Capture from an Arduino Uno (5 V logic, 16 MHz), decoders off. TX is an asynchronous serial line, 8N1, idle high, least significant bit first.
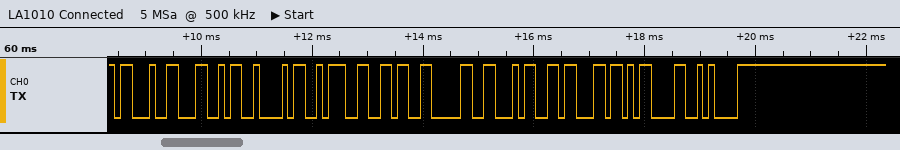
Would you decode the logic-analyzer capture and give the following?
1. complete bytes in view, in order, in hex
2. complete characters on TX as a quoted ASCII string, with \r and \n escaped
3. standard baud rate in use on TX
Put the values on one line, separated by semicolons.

23 4C 42 3A 36 30 34 63 0D 0A; "#LB:604c\r\n"; 9600 baud
